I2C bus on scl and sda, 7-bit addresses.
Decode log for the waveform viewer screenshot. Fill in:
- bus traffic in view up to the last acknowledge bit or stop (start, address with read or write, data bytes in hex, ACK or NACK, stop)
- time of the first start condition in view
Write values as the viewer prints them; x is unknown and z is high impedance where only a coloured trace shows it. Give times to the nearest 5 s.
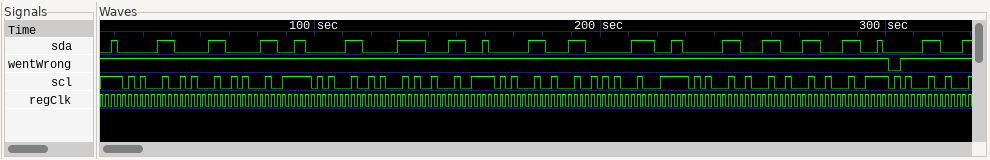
start, address 12 write NACK, stop, start, address 13 write NACK, stop, start, address 14 write NACK, stop, start, address 15 write NACK, stop
30 s
